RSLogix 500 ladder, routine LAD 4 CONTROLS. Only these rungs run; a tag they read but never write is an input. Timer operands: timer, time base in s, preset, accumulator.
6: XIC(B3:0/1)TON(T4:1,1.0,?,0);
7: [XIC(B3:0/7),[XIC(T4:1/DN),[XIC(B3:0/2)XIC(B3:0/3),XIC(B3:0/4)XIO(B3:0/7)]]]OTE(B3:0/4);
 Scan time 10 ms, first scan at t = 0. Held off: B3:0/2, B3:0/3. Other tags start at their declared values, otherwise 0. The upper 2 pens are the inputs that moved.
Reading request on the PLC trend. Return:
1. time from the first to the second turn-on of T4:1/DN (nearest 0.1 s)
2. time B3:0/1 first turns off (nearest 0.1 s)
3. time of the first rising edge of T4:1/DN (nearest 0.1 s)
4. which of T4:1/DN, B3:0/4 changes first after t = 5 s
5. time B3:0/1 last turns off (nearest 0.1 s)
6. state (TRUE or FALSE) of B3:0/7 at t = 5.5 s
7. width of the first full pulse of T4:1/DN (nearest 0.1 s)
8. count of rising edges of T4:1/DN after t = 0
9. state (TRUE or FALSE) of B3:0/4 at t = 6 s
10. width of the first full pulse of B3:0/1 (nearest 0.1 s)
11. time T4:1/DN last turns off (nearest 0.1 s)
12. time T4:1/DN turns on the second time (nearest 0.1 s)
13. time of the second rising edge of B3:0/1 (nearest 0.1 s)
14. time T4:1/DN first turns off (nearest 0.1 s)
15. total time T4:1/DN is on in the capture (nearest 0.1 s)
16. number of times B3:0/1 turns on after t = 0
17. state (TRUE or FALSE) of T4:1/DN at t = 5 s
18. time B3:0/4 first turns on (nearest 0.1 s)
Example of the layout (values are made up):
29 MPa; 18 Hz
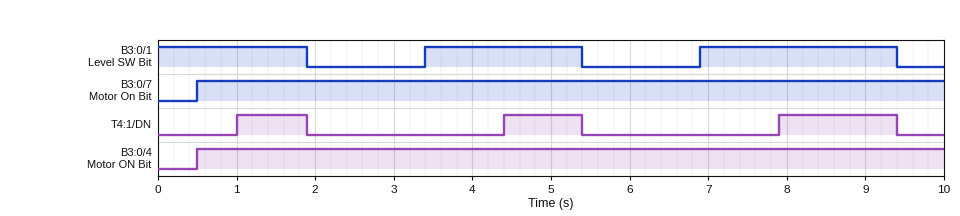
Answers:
3.4 s; 1.9 s; 1.0 s; T4:1/DN; 9.4 s; TRUE; 0.9 s; 3; TRUE; 2.0 s; 9.4 s; 4.4 s; 6.9 s; 1.9 s; 3.4 s; 2; TRUE; 0.5 s
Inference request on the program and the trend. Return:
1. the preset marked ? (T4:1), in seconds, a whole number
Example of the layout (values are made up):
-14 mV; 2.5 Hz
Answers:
1 s
